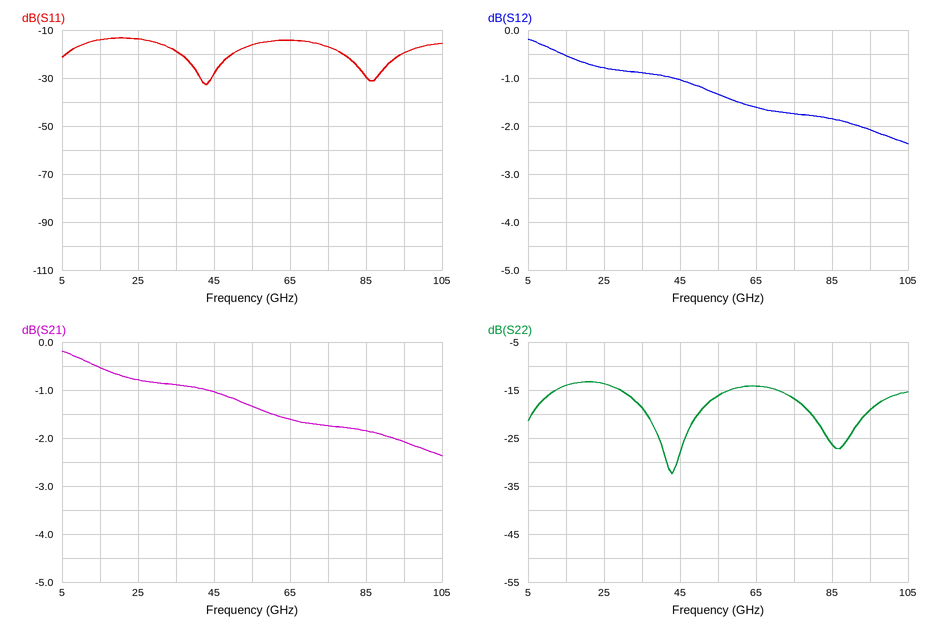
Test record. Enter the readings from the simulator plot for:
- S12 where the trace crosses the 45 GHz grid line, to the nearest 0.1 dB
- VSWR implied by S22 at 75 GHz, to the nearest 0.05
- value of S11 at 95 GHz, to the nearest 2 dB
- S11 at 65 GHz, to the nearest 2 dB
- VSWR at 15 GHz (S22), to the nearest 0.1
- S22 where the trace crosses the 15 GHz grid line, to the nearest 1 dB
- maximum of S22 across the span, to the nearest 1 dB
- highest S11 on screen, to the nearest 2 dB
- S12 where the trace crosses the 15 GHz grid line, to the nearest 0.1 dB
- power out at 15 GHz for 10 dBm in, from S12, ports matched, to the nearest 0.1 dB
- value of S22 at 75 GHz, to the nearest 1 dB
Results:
-1.0 dB
1.35
-20 dB
-14 dB
1.5
-14 dB
-13 dB
-14 dB
-0.5 dB
9.5 dBm
-17 dB
